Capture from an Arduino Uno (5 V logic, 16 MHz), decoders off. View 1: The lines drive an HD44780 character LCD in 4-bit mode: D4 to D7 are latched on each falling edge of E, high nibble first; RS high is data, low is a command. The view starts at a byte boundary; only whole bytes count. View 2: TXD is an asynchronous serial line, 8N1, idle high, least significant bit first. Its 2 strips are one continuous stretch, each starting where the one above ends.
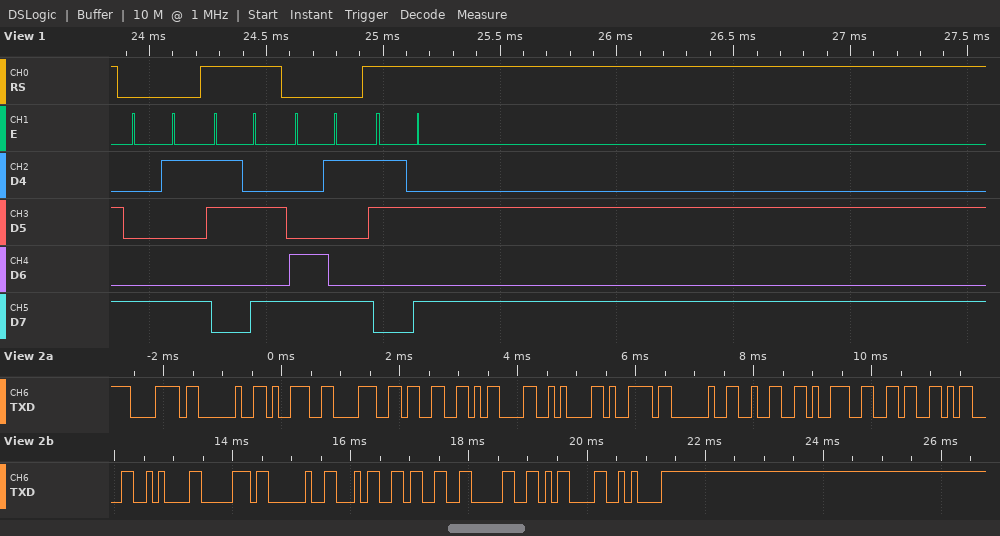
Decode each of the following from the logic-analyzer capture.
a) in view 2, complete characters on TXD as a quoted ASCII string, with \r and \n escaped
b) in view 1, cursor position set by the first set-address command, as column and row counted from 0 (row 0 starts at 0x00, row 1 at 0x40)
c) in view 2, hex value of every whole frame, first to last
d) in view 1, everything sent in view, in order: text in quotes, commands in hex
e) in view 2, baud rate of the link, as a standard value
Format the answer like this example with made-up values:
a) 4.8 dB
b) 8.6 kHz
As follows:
a) "x 983\r\ny 296\r\np 430\r\n"
b) column 9, row 0
c) 78 20 39 38 33 0D 0A 79 20 32 39 36 0D 0A 70 20 34 33 30 0D 0A
d) 0x89 ":" 0xC9 ":"
e) 9600 baud
